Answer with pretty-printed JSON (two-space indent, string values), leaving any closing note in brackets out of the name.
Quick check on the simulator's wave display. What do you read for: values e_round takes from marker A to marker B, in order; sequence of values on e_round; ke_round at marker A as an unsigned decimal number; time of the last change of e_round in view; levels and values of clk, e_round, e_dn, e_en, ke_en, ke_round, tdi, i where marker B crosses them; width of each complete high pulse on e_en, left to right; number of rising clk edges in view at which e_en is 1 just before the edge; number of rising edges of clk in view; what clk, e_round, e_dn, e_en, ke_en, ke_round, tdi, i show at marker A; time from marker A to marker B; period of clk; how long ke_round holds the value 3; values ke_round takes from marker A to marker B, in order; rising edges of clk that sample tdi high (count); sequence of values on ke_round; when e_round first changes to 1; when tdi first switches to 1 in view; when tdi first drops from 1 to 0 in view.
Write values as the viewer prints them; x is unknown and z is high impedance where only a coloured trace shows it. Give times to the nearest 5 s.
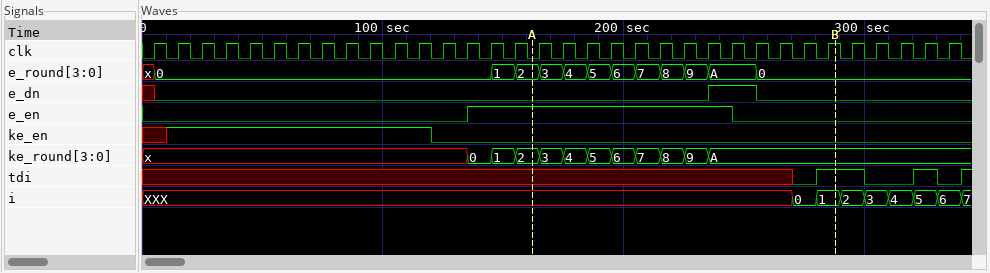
{
  "values e_round takes from marker A to marker B, in order": "2, 3, 4, 5, 6, 7, 8, 9, A, 0",
  "sequence of values on e_round": "x, 0, 1, 2, 3, 4, 5, 6, 7, 8, 9, A, 0",
  "ke_round at marker A as an unsigned decimal number": "2",
  "time of the last change of e_round in view": "255 s",
  "levels and values of clk, e_round, e_dn, e_en, ke_en, ke_round, tdi, i where marker B crosses them": "clk=1, e_round=0, e_dn=0, e_en=0, ke_en=0, ke_round=A, tdi=1, i=1",
  "width of each complete high pulse on e_en, left to right": "110 s",
  "number of rising clk edges in view at which e_en is 1 just before the edge": "11",
  "number of rising edges of clk in view": "34",
  "what clk, e_round, e_dn, e_en, ke_en, ke_round, tdi, i show at marker A": "clk=0, e_round=2, e_dn=0, e_en=1, ke_en=0, ke_round=2, tdi=x, i=XXX",
  "time from marker A to marker B": "125 s",
  "period of clk": "10 s",
  "how long ke_round holds the value 3": "10 s",
  "values ke_round takes from marker A to marker B, in order": "2, 3, 4, 5, 6, 7, 8, 9, A",
  "rising edges of clk that sample tdi high": "3",
  "sequence of values on ke_round": "x, 0, 1, 2, 3, 4, 5, 6, 7, 8, 9, A",
  "when e_round first changes to 1": "145 s",
  "when tdi first switches to 1 in view": "280 s",
  "when tdi first drops from 1 to 0 in view": "300 s"
}
